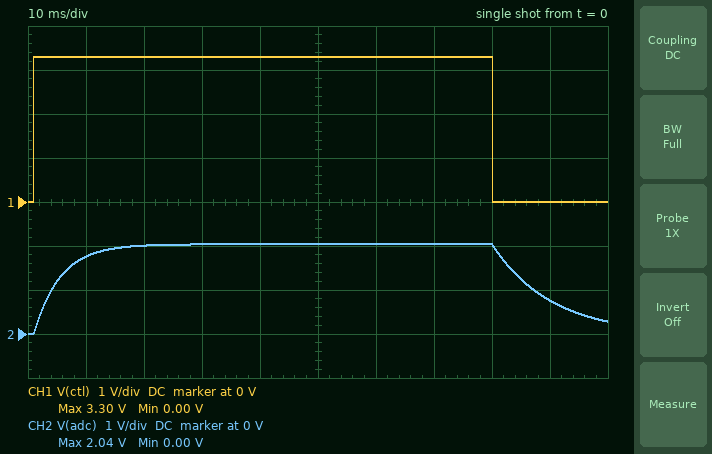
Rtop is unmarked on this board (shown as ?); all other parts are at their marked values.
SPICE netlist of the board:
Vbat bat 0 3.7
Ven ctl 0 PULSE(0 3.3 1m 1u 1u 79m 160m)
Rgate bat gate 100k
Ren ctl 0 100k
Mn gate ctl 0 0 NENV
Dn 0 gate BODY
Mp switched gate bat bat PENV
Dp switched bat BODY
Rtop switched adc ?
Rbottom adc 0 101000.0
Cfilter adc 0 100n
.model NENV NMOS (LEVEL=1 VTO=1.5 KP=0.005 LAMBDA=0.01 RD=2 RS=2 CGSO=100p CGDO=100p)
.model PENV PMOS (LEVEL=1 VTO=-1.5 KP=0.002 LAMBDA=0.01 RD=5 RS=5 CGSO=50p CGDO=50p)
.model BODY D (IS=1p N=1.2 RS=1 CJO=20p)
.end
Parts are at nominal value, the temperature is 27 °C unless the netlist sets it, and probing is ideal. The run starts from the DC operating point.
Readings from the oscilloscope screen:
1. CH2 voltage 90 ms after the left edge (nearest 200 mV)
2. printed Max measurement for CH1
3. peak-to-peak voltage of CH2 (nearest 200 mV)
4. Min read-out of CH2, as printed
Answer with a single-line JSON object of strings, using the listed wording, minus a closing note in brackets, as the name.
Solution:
{"CH2 voltage 90 ms after the left edge": "800 mV", "printed Max measurement for CH1": "3.30 V", "peak-to-peak voltage of CH2": "2.0 V", "Min read-out of CH2, as printed": "0.00 V"}
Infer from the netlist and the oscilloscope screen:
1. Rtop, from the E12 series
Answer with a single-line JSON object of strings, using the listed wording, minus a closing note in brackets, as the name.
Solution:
{"Rtop, from the E12 series": "82 kΩ"}
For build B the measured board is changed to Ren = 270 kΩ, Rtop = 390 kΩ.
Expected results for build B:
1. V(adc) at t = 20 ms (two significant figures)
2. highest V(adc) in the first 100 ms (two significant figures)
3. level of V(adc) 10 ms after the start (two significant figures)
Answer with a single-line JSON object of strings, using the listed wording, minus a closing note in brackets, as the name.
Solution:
{"V(adc) at t = 20 ms": "690 mV", "highest V(adc) in the first 100 ms": "760 mV", "level of V(adc) 10 ms after the start": "510 mV"}
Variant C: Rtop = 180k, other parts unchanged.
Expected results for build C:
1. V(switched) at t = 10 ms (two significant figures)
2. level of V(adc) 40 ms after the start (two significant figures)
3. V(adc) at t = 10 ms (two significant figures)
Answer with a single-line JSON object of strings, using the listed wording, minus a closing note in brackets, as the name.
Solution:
{"V(switched) at t = 10 ms": "3.7 V", "level of V(adc) 40 ms after the start": "1.3 V", "V(adc) at t = 10 ms": "1.0 V"}
